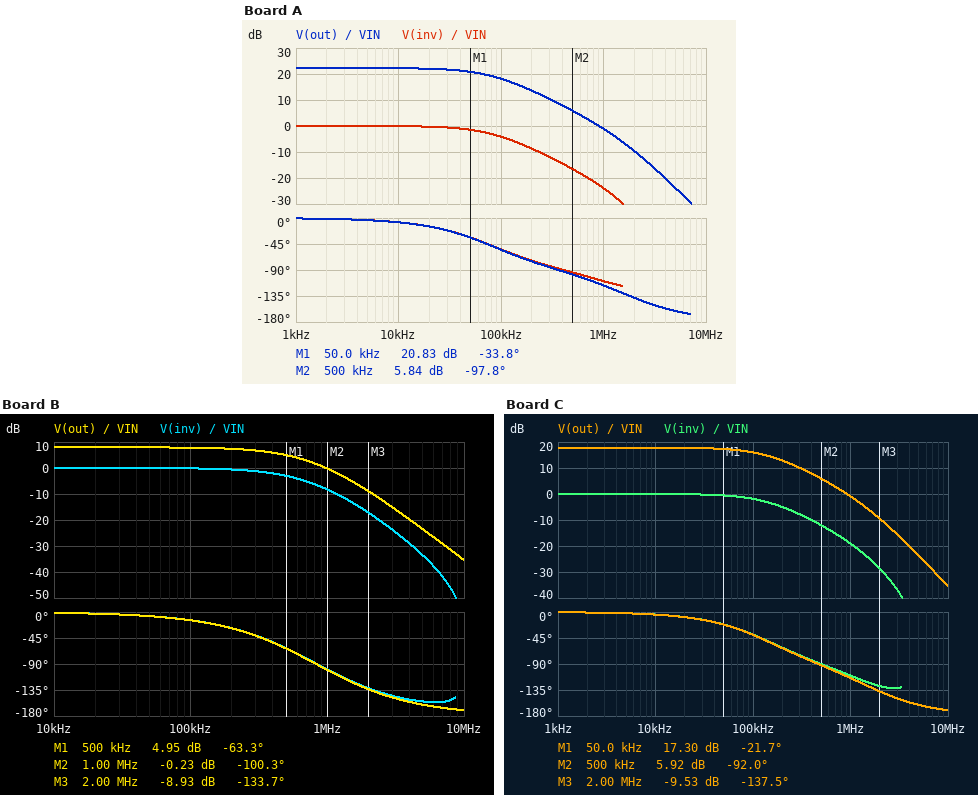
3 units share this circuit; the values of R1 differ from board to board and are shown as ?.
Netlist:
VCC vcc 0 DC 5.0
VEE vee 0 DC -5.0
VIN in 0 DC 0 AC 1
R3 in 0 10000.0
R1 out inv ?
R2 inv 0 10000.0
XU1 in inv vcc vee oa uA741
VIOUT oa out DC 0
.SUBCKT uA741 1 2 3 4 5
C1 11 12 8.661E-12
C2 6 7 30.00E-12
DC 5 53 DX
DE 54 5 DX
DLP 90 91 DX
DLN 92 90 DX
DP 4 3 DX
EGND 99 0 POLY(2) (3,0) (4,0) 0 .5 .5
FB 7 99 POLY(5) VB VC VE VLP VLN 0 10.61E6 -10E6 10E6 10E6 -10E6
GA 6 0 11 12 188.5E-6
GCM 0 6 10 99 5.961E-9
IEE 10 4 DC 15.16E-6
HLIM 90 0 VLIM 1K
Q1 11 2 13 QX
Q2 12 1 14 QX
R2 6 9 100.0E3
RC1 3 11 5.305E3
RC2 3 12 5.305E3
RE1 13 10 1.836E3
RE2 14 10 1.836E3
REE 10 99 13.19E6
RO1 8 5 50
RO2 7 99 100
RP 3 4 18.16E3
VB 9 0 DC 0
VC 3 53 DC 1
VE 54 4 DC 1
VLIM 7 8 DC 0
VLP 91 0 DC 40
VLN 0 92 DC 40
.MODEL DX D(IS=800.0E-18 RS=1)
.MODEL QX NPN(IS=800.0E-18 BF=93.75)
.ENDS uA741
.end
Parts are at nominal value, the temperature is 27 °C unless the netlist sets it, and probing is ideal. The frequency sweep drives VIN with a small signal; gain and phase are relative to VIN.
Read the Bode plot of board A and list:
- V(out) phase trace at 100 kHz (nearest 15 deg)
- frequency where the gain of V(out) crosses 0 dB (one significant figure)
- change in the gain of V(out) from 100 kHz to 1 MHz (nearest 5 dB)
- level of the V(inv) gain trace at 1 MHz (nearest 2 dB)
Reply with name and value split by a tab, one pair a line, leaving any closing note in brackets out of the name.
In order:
V(out) phase trace at 100 kHz	-60 deg
frequency where the gain of V(out) crosses 0 dB	900 kHz
change in the gain of V(out) from 100 kHz to 1 MHz	-20 dB
level of the V(inv) gain trace at 1 MHz	-24 dB
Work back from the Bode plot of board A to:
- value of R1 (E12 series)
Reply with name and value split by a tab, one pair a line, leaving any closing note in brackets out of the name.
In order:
value of R1	120 kΩ
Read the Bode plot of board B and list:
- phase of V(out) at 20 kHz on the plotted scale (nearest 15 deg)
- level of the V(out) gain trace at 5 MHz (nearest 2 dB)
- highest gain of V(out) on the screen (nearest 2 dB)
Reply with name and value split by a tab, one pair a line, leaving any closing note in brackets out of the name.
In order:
phase of V(out) at 20 kHz on the plotted scale	0 deg
level of the V(out) gain trace at 5 MHz	-24 dB
highest gain of V(out) on the screen	8 dB
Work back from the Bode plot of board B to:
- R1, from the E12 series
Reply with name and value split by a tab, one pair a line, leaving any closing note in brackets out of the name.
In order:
R1, from the E12 series	15 kΩ
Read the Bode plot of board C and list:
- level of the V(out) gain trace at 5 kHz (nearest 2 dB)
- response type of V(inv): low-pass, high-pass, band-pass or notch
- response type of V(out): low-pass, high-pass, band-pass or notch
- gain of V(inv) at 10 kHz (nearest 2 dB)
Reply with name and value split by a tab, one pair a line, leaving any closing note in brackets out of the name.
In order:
level of the V(out) gain trace at 5 kHz	18 dB
response type of V(inv): low-pass, high-pass, band-pass or notch	low-pass
response type of V(out): low-pass, high-pass, band-pass or notch	low-pass
gain of V(inv) at 10 kHz	0 dB
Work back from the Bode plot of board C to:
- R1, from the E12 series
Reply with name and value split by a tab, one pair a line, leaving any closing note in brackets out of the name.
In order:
R1, from the E12 series	68 kΩ
